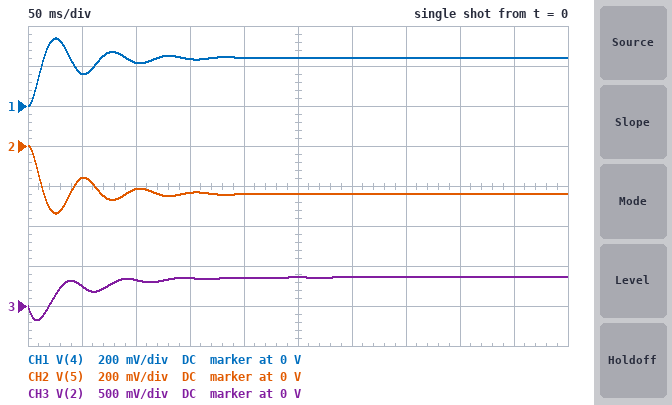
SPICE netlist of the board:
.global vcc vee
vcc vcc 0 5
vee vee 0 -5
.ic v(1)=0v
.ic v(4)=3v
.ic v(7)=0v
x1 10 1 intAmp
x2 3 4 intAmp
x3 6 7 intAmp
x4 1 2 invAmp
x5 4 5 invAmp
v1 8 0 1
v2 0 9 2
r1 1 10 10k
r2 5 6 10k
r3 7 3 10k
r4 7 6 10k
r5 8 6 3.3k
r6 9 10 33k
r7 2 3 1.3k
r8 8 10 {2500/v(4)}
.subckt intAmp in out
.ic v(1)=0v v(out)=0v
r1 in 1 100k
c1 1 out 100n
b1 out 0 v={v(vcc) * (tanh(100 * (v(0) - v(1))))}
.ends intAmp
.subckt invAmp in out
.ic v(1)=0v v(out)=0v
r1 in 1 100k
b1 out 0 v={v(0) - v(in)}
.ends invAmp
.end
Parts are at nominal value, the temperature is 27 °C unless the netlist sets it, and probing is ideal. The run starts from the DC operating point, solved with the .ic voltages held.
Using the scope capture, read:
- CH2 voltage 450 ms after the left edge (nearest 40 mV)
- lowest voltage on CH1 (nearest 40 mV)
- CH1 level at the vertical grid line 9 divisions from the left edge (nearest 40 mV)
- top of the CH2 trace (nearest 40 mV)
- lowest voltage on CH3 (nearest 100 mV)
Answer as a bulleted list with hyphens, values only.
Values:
- -240 mV
- 0 V
- 240 mV
- 0 V
- -200 mV
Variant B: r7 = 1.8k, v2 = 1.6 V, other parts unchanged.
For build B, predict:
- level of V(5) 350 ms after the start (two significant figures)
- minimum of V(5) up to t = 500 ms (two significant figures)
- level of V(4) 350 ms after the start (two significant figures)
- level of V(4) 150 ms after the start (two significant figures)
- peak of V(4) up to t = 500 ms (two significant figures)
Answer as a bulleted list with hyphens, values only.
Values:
- -250 mV
- -310 mV
- 250 mV
- 240 mV
- 310 mV
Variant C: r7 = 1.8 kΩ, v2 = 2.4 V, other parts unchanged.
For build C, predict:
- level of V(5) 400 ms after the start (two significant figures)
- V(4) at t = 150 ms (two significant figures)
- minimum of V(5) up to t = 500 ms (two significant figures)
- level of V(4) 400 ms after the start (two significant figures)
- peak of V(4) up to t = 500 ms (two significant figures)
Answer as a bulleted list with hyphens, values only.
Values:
- -300 mV
- 310 mV
- -430 mV
- 300 mV
- 430 mV
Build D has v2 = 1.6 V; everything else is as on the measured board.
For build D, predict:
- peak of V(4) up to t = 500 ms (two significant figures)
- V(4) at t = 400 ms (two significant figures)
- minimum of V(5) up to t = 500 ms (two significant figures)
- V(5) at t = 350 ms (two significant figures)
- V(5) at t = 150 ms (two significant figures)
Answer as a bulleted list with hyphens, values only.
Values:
- 280 mV
- 210 mV
- -280 mV
- -210 mV
- -200 mV
